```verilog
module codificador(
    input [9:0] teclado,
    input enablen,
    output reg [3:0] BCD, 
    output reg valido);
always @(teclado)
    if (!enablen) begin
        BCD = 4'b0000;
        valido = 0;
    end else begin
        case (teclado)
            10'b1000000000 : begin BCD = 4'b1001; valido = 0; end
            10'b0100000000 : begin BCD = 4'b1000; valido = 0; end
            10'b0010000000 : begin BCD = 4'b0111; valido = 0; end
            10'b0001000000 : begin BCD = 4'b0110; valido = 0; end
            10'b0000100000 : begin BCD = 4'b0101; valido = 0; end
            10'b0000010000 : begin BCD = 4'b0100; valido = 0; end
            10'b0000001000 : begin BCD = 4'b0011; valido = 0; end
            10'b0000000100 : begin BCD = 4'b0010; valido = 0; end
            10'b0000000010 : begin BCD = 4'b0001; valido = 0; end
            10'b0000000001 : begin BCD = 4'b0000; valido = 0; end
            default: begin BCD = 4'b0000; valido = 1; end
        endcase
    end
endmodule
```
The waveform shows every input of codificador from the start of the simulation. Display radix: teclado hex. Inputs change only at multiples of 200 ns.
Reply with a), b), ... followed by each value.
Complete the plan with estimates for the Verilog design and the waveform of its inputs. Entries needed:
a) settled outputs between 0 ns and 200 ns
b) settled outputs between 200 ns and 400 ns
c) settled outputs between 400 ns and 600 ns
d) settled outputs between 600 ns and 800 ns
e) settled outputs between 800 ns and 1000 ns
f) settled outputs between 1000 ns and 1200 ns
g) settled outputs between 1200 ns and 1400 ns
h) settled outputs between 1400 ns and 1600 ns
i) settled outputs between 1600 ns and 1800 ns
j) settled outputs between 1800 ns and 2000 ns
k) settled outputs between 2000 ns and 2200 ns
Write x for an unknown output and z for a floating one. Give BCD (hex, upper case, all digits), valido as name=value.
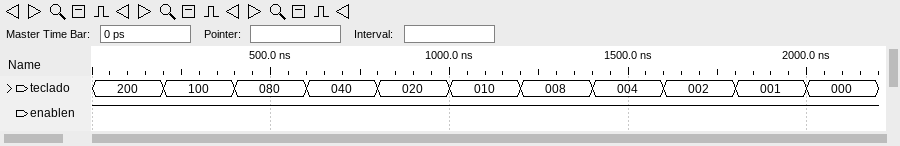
a) BCD=9, valido=0
b) BCD=8, valido=0
c) BCD=7, valido=0
d) BCD=6, valido=0
e) BCD=5, valido=0
f) BCD=4, valido=0
g) BCD=3, valido=0
h) BCD=2, valido=0
i) BCD=1, valido=0
j) BCD=0, valido=0
k) BCD=0, valido=1
